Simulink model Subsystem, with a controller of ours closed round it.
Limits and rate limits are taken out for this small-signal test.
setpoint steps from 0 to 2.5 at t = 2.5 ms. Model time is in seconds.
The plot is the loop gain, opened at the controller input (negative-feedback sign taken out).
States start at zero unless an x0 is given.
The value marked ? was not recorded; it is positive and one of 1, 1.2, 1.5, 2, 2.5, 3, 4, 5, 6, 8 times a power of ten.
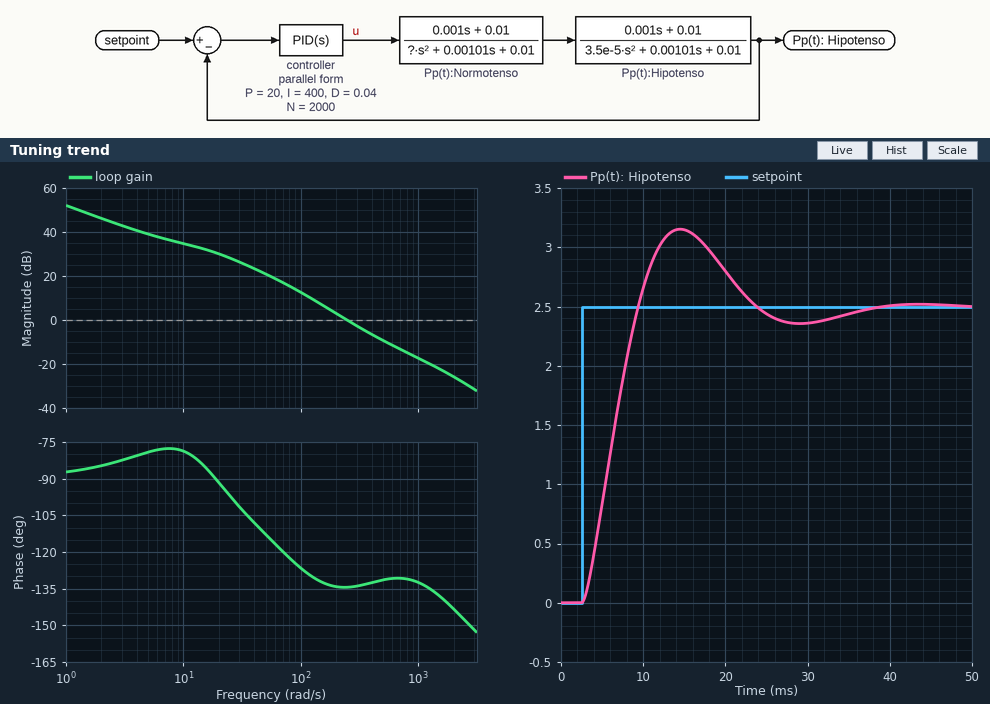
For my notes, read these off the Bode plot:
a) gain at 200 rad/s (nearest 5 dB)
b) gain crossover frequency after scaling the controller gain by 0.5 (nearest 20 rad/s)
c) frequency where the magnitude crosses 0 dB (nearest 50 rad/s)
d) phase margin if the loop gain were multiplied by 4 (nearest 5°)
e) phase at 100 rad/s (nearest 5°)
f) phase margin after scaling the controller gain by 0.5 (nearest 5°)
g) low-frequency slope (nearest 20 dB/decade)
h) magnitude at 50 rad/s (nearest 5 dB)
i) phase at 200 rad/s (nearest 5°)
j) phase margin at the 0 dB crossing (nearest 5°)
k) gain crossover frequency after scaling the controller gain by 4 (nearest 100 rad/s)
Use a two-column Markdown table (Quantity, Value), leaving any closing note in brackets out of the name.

| Quantity | Value |
|---|---|
| gain at 200 rad/s | 5 dB |
| gain crossover frequency after scaling the controller gain by 0.5 | 160 rad/s |
| frequency where the magnitude crosses 0 dB | 250 rad/s |
| phase margin if the loop gain were multiplied by 4 | 50° |
| phase at 100 rad/s | -125° |
| phase margin after scaling the controller gain by 0.5 | 45° |
| low-frequency slope | -20 dB/decade |
| magnitude at 50 rad/s | 20 dB |
| phase at 200 rad/s | -135° |
| phase margin at the 0 dB crossing | 45° |
| gain crossover frequency after scaling the controller gain by 4 | 600 rad/s |
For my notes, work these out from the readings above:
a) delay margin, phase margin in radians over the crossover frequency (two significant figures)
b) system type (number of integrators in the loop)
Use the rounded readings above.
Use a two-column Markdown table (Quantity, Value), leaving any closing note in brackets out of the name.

| Quantity | Value |
|---|---|
| delay margin, phase margin in radians over the crossover frequency | 0.0031 s |
| system type | 1 |
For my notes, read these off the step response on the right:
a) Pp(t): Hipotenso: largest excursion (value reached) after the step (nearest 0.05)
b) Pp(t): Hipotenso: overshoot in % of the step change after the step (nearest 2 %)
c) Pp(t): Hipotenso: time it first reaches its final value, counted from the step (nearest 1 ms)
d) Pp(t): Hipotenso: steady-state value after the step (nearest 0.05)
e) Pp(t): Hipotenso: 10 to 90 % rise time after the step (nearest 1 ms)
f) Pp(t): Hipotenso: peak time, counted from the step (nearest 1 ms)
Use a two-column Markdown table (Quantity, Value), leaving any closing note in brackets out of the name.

| Quantity | Value |
|---|---|
| Pp(t): Hipotenso: largest excursion (value reached) after the step | 3.15 |
| Pp(t): Hipotenso: overshoot in % of the step change after the step | 26 % |
| Pp(t): Hipotenso: time it first reaches its final value, counted from the step | 7 ms |
| Pp(t): Hipotenso: steady-state value after the step | 2.50 |
| Pp(t): Hipotenso: 10 to 90 % rise time after the step | 5 ms |
| Pp(t): Hipotenso: peak time, counted from the step | 12 ms |
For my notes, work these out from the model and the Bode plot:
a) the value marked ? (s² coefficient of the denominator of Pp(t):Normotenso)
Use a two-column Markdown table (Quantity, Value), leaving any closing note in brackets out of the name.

| Quantity | Value |
|---|---|
| the value marked ? (s² coefficient of the denominator of Pp(t):Normotenso) | 1e-05 |
